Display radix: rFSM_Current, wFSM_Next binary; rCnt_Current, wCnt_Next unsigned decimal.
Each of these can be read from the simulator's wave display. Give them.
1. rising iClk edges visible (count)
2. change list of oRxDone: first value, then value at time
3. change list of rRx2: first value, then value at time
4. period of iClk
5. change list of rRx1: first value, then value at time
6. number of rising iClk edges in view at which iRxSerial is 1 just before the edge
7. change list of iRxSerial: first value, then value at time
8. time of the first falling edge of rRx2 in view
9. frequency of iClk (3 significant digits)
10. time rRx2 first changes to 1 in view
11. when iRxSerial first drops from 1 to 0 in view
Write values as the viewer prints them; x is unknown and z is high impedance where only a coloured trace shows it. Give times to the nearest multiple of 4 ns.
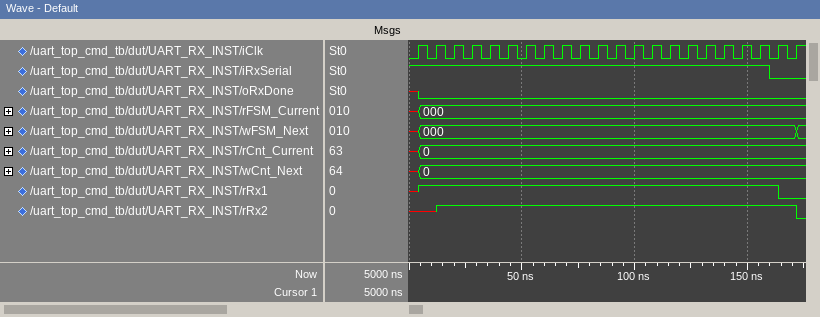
22
x, 0 at 4 ns
x, 1 at 12 ns, 0 at 172 ns
8 ns
x, 1 at 4 ns, 0 at 164 ns
20
1, 0 at 160 ns
172 ns
125 MHz
12 ns
160 ns
